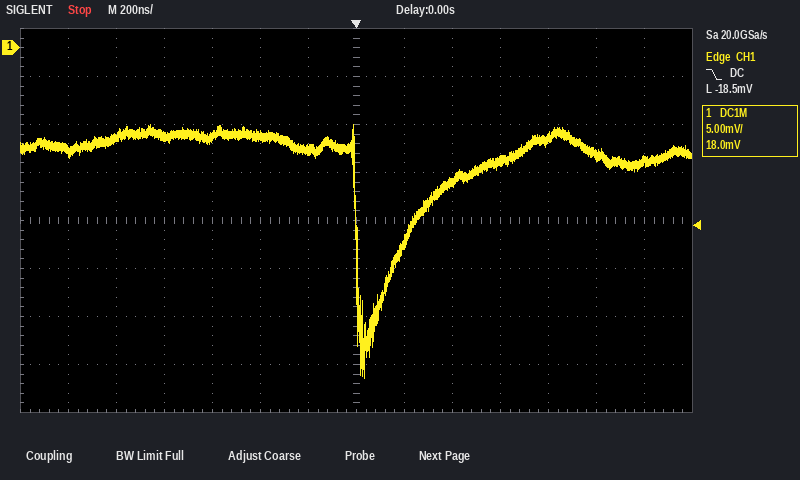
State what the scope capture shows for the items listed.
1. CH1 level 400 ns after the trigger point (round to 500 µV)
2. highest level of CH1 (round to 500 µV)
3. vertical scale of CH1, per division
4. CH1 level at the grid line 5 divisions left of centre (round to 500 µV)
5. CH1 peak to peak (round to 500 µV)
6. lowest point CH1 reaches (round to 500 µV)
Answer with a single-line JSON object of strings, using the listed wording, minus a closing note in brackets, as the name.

{"CH1 level 400 ns after the trigger point": "-14.0 mV", "highest level of CH1": "-8.0 mV", "vertical scale of CH1, per division": "5 mV", "CH1 level at the grid line 5 divisions left of centre": "-9.5 mV", "CH1 peak to peak": "26.5 mV", "lowest point CH1 reaches": "-34.5 mV"}
